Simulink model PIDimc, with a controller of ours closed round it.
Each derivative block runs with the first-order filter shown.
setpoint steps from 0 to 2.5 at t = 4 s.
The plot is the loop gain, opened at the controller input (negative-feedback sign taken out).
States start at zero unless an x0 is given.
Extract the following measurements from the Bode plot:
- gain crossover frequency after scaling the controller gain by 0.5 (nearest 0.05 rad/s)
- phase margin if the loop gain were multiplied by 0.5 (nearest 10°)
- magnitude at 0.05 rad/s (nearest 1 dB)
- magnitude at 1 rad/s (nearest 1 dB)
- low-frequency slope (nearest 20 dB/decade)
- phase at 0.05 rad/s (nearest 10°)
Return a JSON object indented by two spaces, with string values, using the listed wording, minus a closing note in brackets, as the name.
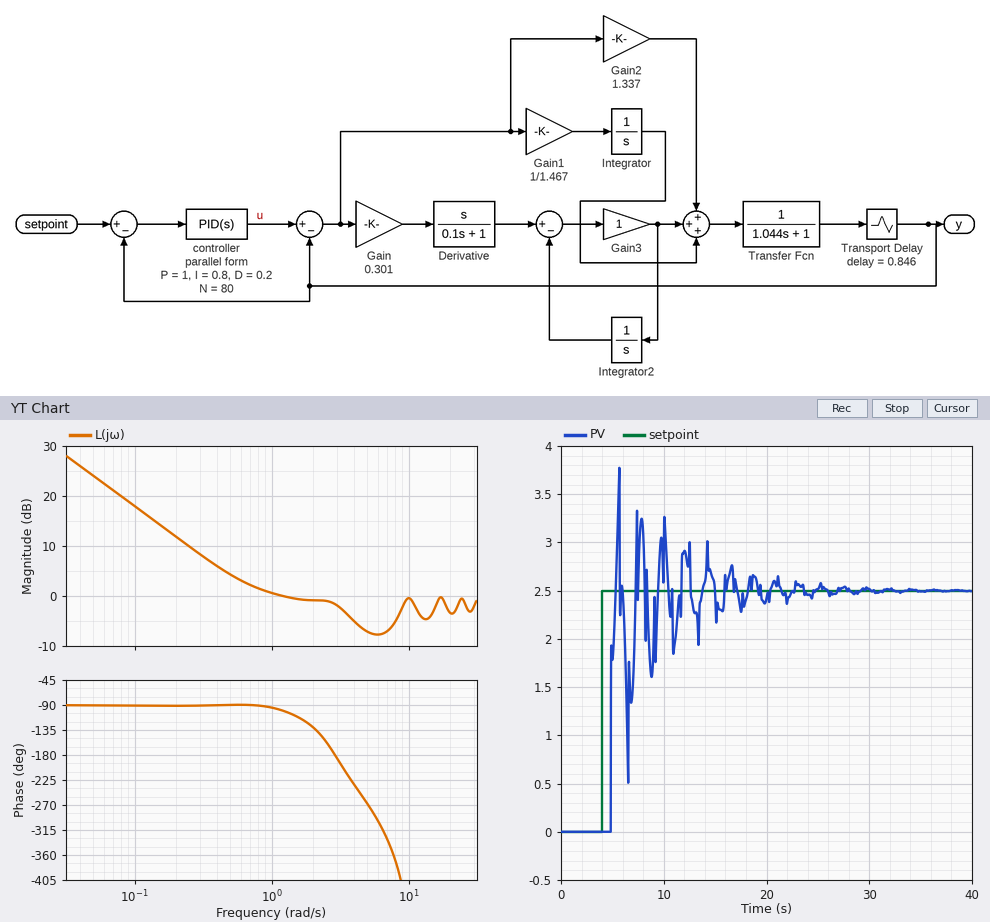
{
  "gain crossover frequency after scaling the controller gain by 0.5": "0.40 rad/s",
  "phase margin if the loop gain were multiplied by 0.5": "90°",
  "magnitude at 0.05 rad/s": "24 dB",
  "magnitude at 1 rad/s": "1 dB",
  "low-frequency slope": "-20 dB/decade",
  "phase at 0.05 rad/s": "-90°"
}
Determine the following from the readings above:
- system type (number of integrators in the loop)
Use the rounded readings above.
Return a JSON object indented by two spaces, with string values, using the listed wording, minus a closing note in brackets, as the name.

{
  "system type": "1"
}
